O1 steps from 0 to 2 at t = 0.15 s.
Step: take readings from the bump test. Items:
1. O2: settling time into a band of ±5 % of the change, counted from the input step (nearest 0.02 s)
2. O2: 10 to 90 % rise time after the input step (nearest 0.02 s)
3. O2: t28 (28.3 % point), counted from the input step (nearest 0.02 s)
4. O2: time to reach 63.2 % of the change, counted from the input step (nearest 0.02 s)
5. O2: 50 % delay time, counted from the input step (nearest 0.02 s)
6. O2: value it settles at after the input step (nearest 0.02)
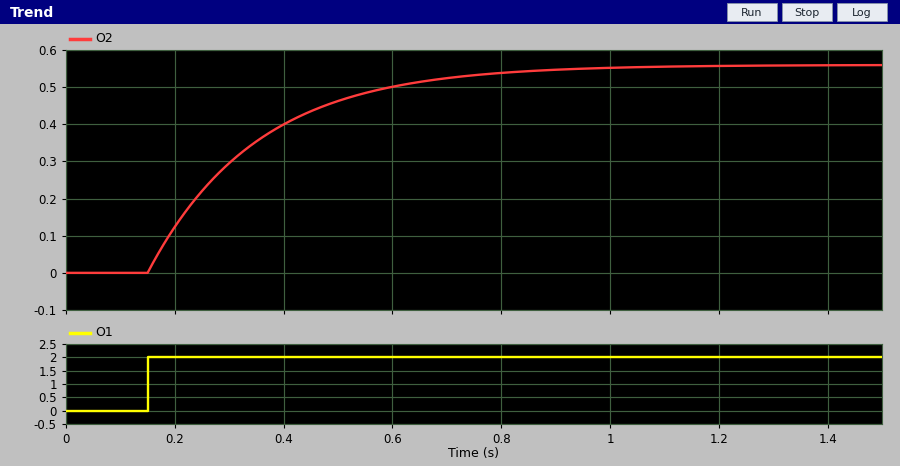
0.60 s
0.44 s
0.06 s
0.20 s
0.14 s
0.56
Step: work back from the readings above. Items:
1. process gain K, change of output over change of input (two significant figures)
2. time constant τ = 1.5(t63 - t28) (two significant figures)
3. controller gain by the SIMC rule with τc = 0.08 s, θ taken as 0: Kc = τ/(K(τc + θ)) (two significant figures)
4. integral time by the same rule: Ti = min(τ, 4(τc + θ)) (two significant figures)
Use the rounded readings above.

0.28
0.21 s
9.4
0.21 s
